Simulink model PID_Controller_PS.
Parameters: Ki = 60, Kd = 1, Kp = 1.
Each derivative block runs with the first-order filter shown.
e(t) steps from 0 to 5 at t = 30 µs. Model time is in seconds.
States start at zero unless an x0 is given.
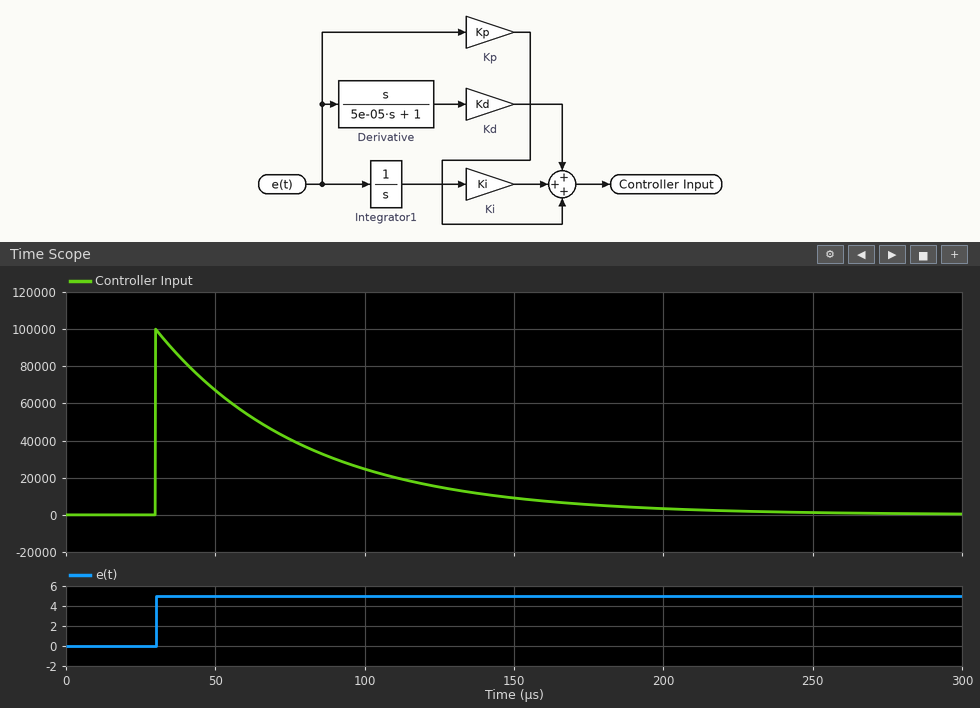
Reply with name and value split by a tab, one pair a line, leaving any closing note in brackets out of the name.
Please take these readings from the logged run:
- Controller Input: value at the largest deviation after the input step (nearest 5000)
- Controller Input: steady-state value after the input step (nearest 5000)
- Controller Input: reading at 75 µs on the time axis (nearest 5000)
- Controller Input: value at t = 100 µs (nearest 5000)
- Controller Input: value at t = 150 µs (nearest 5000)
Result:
Controller Input: value at the largest deviation after the input step	100000
Controller Input: steady-state value after the input step	0
Controller Input: reading at 75 µs on the time axis	40000
Controller Input: value at t = 100 µs	25000
Controller Input: value at t = 150 µs	10000
